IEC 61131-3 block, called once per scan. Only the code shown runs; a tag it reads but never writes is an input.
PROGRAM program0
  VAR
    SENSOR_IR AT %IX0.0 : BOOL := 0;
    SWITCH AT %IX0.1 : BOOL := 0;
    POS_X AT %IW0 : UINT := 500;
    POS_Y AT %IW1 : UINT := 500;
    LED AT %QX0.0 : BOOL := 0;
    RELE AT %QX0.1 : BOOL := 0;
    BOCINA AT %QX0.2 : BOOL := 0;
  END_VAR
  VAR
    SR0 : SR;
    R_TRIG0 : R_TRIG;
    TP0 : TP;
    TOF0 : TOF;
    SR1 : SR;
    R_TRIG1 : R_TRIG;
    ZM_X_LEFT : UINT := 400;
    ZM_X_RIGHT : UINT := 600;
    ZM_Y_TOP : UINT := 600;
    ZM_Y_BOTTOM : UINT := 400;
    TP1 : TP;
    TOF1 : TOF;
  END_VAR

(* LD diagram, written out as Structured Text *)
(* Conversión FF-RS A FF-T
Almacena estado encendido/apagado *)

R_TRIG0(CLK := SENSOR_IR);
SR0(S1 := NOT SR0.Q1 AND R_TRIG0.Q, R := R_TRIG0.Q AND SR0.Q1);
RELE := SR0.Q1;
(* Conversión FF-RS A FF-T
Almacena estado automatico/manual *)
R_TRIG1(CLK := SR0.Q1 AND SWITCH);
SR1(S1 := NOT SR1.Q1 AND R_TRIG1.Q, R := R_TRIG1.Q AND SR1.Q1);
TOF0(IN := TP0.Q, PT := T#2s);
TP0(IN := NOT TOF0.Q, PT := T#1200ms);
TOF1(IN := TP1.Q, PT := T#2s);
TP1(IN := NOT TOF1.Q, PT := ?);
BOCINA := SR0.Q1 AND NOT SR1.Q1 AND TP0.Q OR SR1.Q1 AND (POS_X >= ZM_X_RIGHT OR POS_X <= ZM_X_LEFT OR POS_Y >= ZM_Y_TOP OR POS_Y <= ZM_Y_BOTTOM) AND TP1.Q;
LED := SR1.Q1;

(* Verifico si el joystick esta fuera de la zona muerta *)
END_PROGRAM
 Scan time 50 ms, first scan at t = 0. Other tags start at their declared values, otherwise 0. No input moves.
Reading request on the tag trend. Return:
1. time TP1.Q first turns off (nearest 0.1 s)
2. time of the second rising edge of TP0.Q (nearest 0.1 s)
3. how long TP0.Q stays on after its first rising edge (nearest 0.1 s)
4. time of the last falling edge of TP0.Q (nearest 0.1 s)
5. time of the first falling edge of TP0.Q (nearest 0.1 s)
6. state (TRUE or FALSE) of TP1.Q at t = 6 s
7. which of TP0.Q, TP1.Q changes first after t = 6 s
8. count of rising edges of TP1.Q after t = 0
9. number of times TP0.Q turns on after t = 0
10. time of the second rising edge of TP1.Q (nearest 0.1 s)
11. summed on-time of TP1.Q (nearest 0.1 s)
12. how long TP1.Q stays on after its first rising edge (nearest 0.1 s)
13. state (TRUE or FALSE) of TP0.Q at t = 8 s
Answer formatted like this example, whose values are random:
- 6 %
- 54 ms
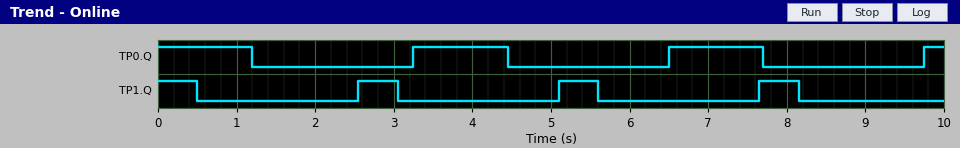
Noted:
- 0.5 s
- 6.5 s
- 1.2 s
- 7.7 s
- 1.2 s
- FALSE
- TP0.Q
- 3
- 3
- 5.1 s
- 2.0 s
- 0.5 s
- FALSE
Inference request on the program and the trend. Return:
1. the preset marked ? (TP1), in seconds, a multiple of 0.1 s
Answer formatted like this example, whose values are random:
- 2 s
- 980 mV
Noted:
- 0.5 s
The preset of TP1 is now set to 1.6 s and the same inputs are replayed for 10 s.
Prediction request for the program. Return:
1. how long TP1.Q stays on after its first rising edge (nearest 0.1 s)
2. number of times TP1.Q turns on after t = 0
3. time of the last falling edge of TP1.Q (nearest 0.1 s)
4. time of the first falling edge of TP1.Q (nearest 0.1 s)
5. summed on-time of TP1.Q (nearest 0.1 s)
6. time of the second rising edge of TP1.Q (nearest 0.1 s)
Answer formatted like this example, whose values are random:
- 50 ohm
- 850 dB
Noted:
- 1.6 s
- 2
- 8.9 s
- 1.6 s
- 4.8 s
- 7.3 s
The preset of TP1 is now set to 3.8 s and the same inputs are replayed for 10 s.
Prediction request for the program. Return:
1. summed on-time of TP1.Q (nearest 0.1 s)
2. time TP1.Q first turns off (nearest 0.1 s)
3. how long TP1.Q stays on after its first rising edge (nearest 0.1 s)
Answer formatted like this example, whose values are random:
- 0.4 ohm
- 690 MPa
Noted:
- 7.6 s
- 3.8 s
- 3.8 s
